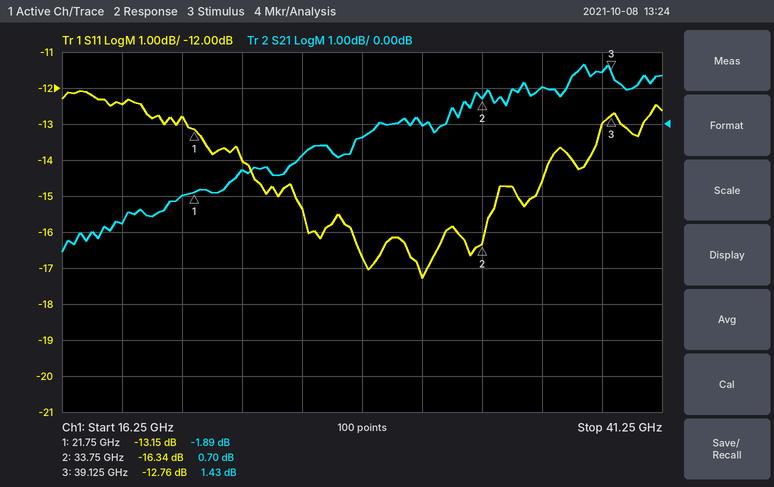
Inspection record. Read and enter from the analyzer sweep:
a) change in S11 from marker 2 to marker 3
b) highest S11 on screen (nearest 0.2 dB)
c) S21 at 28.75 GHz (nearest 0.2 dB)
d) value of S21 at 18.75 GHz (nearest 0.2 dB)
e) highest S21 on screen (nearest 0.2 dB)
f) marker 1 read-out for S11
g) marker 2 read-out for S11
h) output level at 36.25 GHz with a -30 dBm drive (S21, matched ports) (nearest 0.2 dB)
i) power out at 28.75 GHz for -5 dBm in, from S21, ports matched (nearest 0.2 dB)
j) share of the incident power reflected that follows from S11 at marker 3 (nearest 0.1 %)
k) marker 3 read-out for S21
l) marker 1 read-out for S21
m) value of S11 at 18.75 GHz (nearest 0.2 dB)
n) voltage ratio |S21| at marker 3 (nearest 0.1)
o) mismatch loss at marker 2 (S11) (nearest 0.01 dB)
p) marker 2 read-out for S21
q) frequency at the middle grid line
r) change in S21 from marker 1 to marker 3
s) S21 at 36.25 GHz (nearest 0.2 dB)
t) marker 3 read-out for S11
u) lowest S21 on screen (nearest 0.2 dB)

3.58 dB
-12.0 dB
-0.4 dB
-2.8 dB
1.6 dB
-13.15 dB
-16.34 dB
-29.0 dBm
-5.4 dBm
5.3 %
1.43 dB
-1.89 dB
-12.4 dB
1.2
0.10 dB
0.70 dB
28.75 GHz
3.32 dB
1.0 dB
-12.76 dB
-3.6 dB
